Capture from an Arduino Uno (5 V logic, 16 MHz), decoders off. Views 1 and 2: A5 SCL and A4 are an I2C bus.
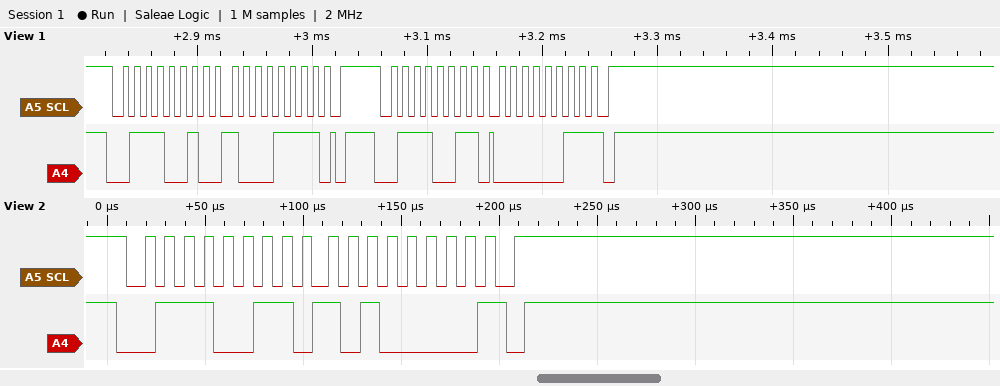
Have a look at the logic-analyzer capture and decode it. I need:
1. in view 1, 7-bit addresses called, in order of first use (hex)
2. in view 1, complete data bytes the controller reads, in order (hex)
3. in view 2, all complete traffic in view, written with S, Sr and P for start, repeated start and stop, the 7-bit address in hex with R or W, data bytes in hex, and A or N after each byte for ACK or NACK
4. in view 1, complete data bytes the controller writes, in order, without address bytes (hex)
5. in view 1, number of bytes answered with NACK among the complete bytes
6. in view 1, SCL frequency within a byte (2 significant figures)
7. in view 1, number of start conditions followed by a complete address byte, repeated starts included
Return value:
0x39
03
S 39R A A0 N P
8F
1
100 kHz
2
